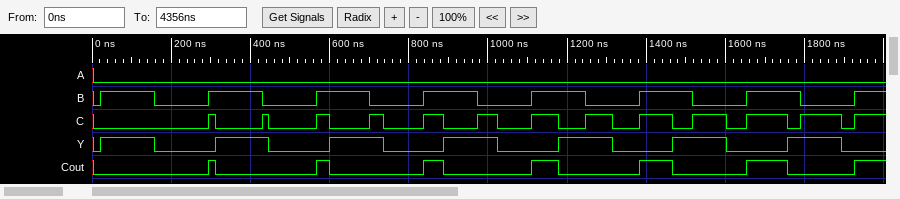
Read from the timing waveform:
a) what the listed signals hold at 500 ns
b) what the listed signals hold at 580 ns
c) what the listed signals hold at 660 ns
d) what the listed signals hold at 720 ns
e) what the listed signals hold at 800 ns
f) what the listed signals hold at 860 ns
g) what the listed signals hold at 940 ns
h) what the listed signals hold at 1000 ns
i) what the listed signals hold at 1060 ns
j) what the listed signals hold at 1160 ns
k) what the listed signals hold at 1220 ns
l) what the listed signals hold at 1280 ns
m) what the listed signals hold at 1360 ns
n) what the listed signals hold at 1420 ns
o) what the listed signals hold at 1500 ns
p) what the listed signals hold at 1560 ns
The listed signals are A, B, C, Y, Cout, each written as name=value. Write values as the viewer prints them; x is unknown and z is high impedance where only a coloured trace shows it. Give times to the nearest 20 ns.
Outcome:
A=0, B=0, C=0, Y=0, Cout=0
A=0, B=1, C=1, Y=0, Cout=1
A=0, B=1, C=0, Y=1, Cout=0
A=0, B=0, C=1, Y=1, Cout=0
A=0, B=0, C=0, Y=0, Cout=0
A=0, B=1, C=1, Y=0, Cout=1
A=0, B=1, C=0, Y=1, Cout=0
A=0, B=0, C=1, Y=1, Cout=0
A=0, B=0, C=0, Y=0, Cout=0
A=0, B=1, C=1, Y=0, Cout=1
A=0, B=1, C=0, Y=1, Cout=0
A=0, B=0, C=1, Y=1, Cout=0
A=0, B=0, C=0, Y=0, Cout=0
A=0, B=1, C=1, Y=0, Cout=1
A=0, B=1, C=0, Y=1, Cout=0
A=0, B=0, C=1, Y=1, Cout=0
